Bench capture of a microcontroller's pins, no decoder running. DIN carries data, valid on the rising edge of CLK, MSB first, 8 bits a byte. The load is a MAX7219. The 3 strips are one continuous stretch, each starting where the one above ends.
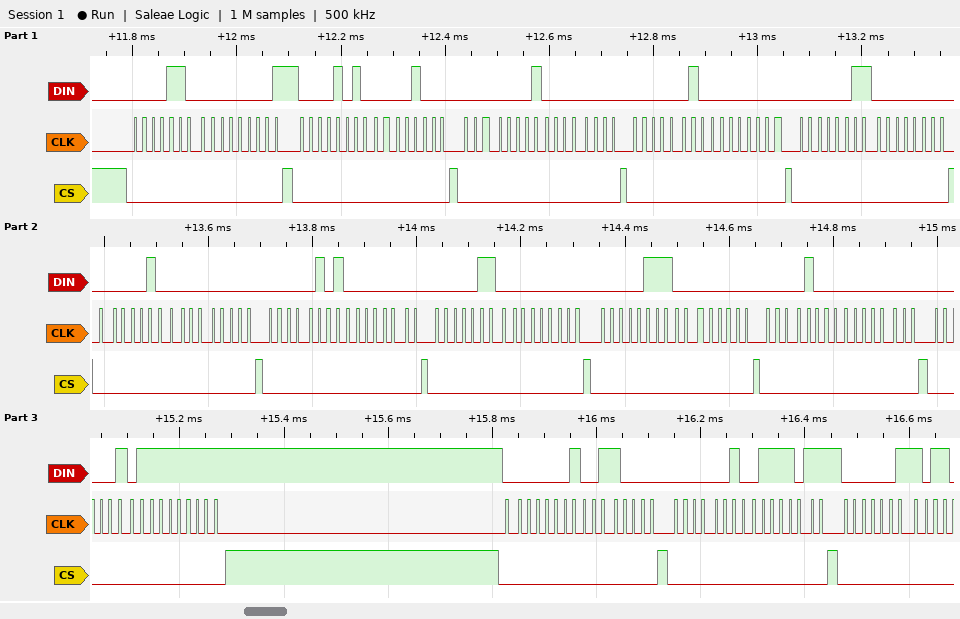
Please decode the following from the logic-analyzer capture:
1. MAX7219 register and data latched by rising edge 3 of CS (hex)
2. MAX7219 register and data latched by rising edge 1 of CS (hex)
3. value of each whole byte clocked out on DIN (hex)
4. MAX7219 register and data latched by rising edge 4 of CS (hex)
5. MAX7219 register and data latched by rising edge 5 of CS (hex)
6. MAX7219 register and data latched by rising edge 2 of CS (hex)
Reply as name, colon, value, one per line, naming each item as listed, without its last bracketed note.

MAX7219 register and data latched by rising edge 3 of CS: register 0x1, data 0x00
MAX7219 register and data latched by rising edge 1 of CS: register 0xC, data 0x01
value of each whole byte clocked out on DIN: 0C 01 0A 08 01 00 02 00 03 00 04 00 05 00 06 00 07 00 08 00 05 FF 01 30 02 7B 03
MAX7219 register and data latched by rising edge 4 of CS: register 0x2, data 0x00
MAX7219 register and data latched by rising edge 5 of CS: register 0x3, data 0x00
MAX7219 register and data latched by rising edge 2 of CS: register 0xA, data 0x08
